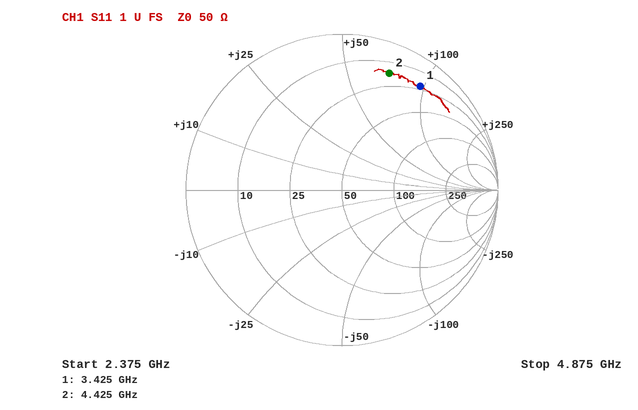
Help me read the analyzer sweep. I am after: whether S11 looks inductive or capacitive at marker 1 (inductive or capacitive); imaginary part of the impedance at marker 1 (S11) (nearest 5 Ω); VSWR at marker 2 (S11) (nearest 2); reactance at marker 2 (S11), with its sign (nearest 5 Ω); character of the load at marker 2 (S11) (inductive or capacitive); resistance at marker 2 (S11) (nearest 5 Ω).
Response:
inductive
+95 Ω
10
+70 Ω
inductive
15 Ω
